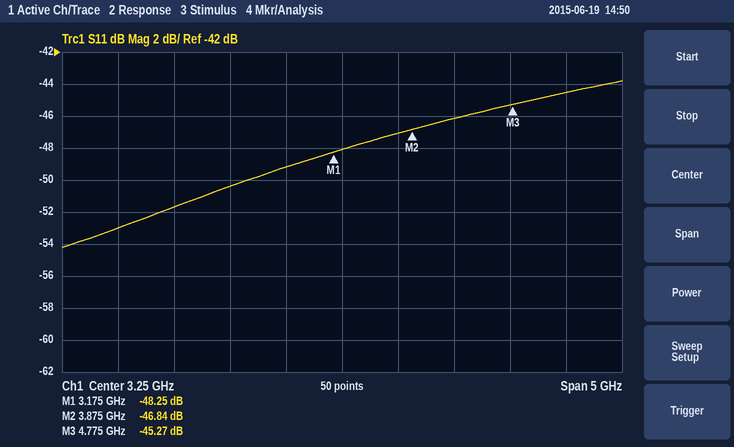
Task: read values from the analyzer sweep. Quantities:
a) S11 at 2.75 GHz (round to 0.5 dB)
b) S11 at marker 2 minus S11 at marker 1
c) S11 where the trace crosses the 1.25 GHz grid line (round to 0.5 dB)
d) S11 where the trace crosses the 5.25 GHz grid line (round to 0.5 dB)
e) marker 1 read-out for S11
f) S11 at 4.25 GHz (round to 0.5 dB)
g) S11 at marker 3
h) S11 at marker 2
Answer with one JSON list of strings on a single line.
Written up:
["-49.0 dB", "1.41 dB", "-53.0 dB", "-44.5 dB", "-48.25 dB", "-46.0 dB", "-45.27 dB", "-46.84 dB"]
